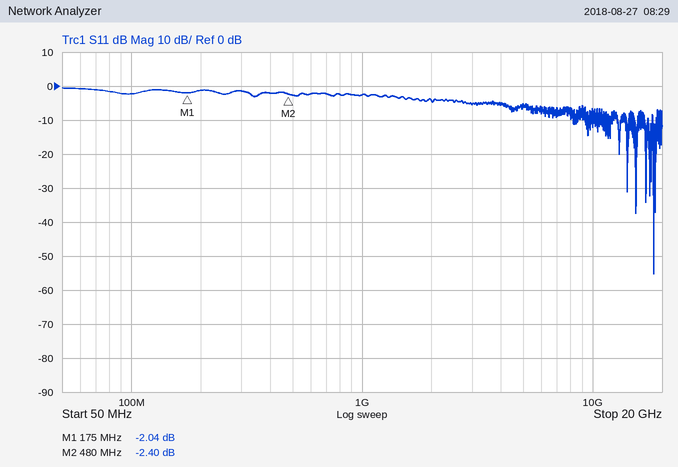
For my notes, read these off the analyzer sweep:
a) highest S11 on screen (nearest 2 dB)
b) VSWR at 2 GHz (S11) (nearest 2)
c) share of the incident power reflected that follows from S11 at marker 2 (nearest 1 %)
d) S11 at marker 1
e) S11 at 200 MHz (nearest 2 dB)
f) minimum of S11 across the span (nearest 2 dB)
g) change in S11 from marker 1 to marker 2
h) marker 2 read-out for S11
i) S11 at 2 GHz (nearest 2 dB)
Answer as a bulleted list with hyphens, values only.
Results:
- 0 dB
- 4
- 58 %
- -2.04 dB
- -2 dB
- -56 dB
- -0.36 dB
- -2.40 dB
- -4 dB
